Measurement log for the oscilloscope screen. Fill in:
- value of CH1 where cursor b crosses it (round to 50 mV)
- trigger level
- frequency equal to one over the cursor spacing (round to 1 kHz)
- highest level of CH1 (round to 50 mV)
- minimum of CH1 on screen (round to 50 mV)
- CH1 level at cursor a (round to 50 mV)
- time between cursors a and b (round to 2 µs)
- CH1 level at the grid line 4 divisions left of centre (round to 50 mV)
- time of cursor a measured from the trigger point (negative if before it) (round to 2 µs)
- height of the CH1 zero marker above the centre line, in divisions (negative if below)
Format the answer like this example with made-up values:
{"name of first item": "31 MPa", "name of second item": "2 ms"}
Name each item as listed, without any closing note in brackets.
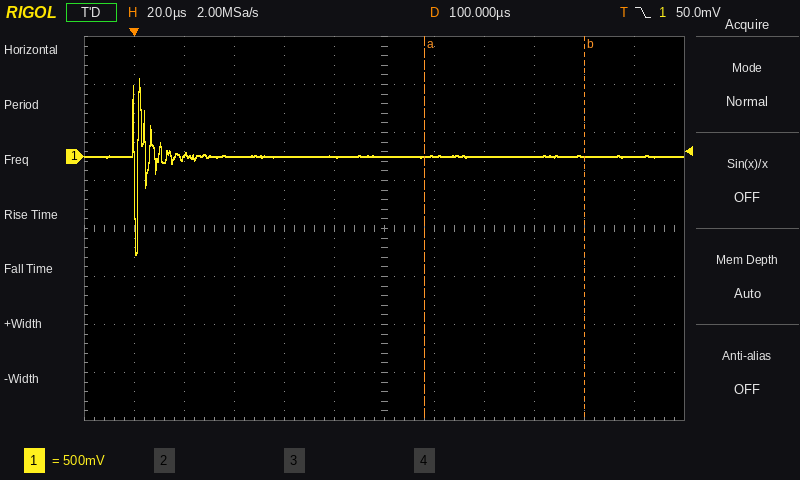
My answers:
{"value of CH1 where cursor b crosses it": "0 mV", "trigger level": "50.0 mV", "frequency equal to one over the cursor spacing": "16 kHz", "highest level of CH1": "800 mV", "minimum of CH1 on screen": "-1.00 V", "CH1 level at cursor a": "0 mV", "time between cursors a and b": "64 µs", "CH1 level at the grid line 4 divisions left of centre": "0 mV", "time of cursor a measured from the trigger point (negative if before it)": "+116 µs", "height of the CH1 zero marker above the centre line, in divisions": "+1.5 div"}
